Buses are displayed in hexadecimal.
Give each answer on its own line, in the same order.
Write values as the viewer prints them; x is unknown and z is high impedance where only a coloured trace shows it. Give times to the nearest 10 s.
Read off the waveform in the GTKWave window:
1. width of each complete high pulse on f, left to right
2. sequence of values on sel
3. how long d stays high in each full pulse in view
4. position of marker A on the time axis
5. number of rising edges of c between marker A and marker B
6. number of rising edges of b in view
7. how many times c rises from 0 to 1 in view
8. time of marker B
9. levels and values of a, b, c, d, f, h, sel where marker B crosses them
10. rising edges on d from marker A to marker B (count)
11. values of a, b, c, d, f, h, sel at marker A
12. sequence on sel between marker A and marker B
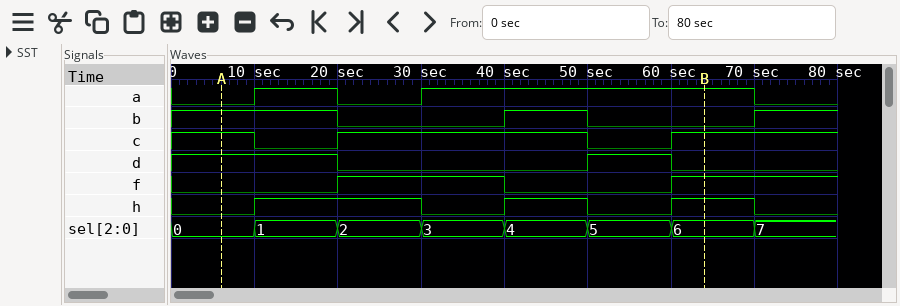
20 s
0, 1, 2, 3, 4, 5, 6, 7
10 s
10 s
2
2
2
60 s
a=1, b=0, c=1, d=0, f=1, h=1, sel=6
1
a=0, b=1, c=1, d=1, f=0, h=0, sel=0
0, 1, 2, 3, 4, 5, 6
